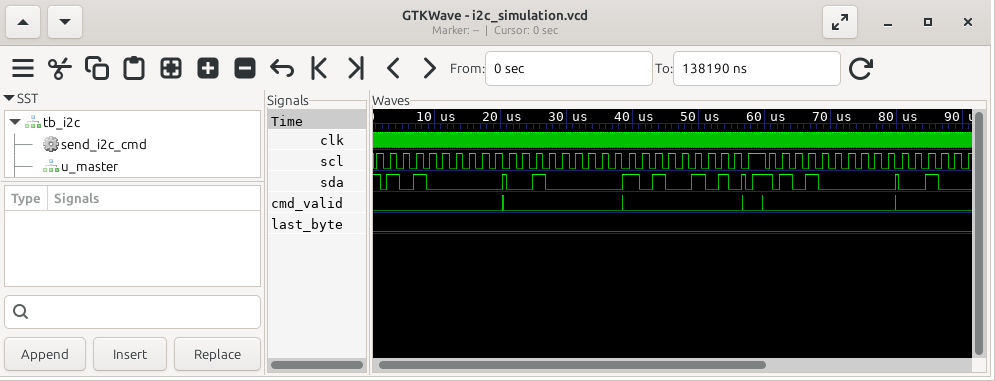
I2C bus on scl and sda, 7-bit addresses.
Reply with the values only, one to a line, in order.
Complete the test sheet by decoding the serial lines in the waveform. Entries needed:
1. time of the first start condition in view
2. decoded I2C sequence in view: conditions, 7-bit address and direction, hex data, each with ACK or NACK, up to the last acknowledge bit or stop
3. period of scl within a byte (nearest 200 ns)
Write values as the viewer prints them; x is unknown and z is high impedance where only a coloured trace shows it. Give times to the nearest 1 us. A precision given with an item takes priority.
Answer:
2 us
start, address 50 write ACK, 20 ACK, A5 ACK, stop, start, address 50 write ACK
2000 ns
